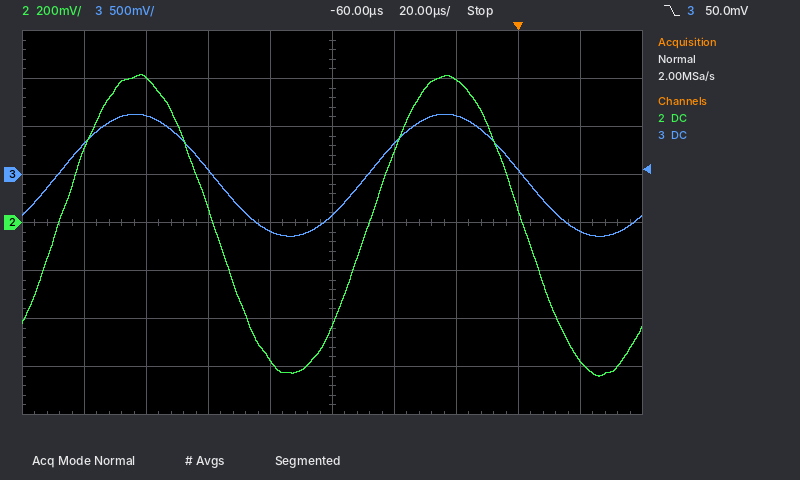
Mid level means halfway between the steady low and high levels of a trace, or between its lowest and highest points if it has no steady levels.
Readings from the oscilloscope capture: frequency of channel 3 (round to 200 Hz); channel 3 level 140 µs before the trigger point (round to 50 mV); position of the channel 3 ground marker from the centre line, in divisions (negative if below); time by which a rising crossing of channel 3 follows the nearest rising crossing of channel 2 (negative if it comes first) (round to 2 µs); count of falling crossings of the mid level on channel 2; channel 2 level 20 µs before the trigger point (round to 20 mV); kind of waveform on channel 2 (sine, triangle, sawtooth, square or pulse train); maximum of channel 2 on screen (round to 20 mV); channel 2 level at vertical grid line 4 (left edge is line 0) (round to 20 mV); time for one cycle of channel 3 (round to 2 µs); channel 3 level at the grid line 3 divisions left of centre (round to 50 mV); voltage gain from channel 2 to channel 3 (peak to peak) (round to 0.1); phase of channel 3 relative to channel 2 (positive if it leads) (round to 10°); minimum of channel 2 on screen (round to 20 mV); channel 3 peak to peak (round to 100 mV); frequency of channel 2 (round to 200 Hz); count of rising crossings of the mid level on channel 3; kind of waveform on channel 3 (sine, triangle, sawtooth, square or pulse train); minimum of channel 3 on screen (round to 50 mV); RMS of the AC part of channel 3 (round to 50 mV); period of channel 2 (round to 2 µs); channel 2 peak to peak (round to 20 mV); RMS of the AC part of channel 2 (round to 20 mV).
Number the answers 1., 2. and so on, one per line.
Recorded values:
1. 10.0 kHz
2. 300 mV
3. +1.0 div
4. 0 µs
5. 2
6. 600 mV
7. sine
8. 620 mV
9. -580 mV
10. 100 µs
11. 600 mV
12. 1.0
13. 0°
14. -640 mV
15. 1.30 V
16. 10.0 kHz
17. 2
18. sine
19. -650 mV
20. 450 mV
21. 100 µs
22. 1.26 V
23. 440 mV
